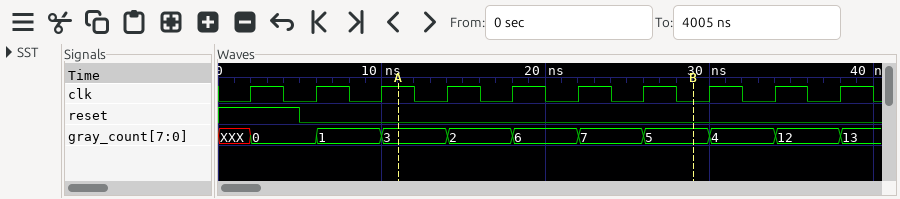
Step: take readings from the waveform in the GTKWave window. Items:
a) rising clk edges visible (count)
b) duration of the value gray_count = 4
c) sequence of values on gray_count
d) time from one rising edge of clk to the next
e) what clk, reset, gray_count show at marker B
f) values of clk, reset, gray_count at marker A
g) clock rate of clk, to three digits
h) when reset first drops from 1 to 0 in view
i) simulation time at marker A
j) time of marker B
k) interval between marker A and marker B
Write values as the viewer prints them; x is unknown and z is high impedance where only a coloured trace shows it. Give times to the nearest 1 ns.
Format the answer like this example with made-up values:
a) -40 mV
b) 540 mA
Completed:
a) 10
b) 4 ns
c) XXX, 0, 1, 3, 2, 6, 7, 5, 4, 12, 13
d) 4 ns
e) clk=0, reset=0, gray_count=5
f) clk=1, reset=0, gray_count=3
g) 250 MHz
h) 5 ns
i) 11 ns
j) 29 ns
k) 18 ns
